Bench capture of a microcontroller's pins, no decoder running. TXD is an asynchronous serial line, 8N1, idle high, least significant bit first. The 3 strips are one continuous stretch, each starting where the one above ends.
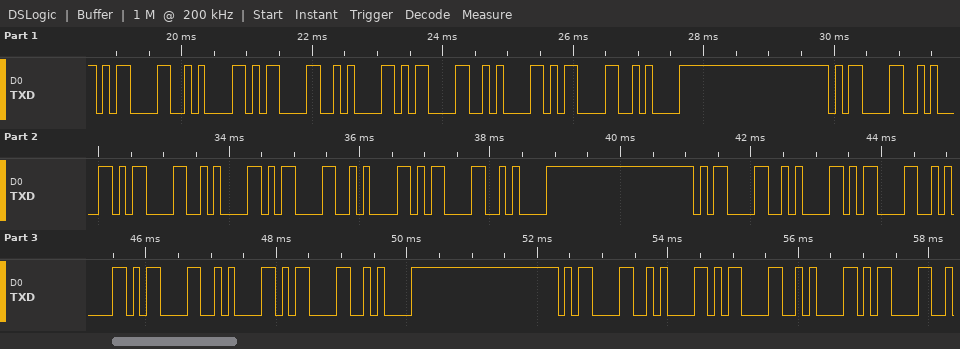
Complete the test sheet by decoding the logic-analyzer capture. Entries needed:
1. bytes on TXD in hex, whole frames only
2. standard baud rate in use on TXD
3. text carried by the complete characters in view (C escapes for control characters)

0D 0A 0D 0A 0D 0A 0D 0A 0D 0A 0D 0A 0D 0A 0D 0A 0D 0A 0D 0A 0D 0A 0D 0A 0D 0A 0D 0A 0D
9600 baud
"\r\n\r\n\r\n\r\n\r\n\r\n\r\n\r\n\r\n\r\n\r\n\r\n\r\n\r\n\r"
